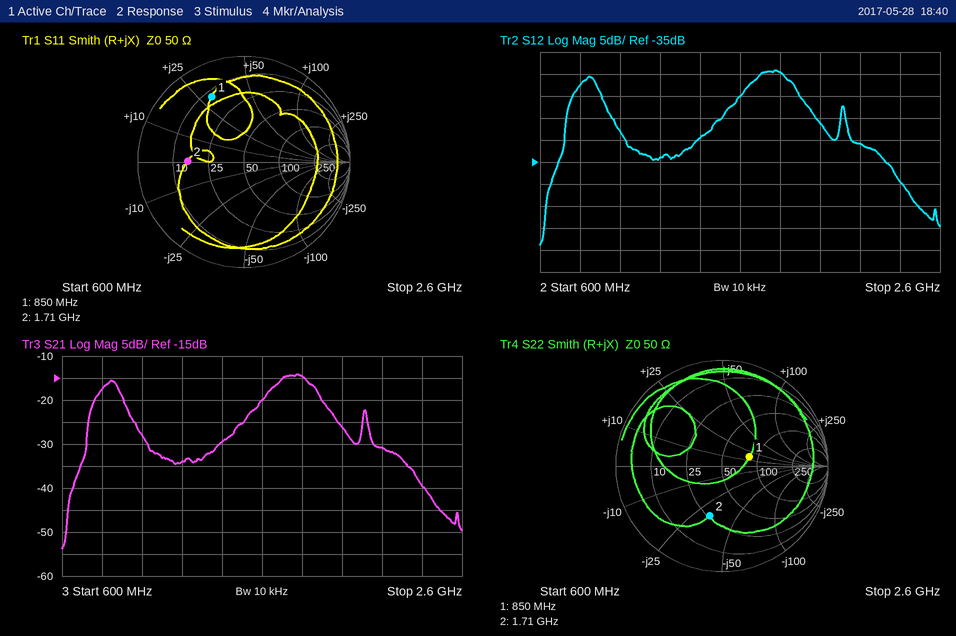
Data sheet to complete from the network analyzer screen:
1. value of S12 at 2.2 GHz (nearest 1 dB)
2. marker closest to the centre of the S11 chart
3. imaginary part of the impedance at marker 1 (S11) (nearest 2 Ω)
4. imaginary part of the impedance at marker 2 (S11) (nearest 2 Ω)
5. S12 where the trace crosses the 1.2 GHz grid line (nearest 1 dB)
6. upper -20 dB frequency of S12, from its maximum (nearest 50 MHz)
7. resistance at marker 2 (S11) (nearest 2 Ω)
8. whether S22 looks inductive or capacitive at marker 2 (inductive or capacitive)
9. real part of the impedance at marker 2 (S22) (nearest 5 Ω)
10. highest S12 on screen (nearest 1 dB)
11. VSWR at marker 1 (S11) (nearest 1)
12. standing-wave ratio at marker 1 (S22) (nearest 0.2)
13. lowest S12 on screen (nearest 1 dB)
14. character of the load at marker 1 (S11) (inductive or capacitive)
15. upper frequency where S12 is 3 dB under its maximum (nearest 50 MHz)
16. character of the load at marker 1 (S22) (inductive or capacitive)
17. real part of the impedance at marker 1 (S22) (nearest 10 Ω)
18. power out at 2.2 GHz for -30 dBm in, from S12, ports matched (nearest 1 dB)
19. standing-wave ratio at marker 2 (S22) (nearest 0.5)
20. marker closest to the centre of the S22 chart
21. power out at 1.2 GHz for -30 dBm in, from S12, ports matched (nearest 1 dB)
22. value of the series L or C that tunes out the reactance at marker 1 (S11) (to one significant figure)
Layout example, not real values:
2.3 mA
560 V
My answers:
-31 dB
marker 2
+30 Ω
0 Ω
-34 dB
2.30 GHz
16 Ω
capacitive
25 Ω
-14 dB
5
1.8
-54 dB
inductive
1.85 GHz
inductive
80 Ω
-61 dBm
3.0
marker 1
-64 dBm
6 pF
